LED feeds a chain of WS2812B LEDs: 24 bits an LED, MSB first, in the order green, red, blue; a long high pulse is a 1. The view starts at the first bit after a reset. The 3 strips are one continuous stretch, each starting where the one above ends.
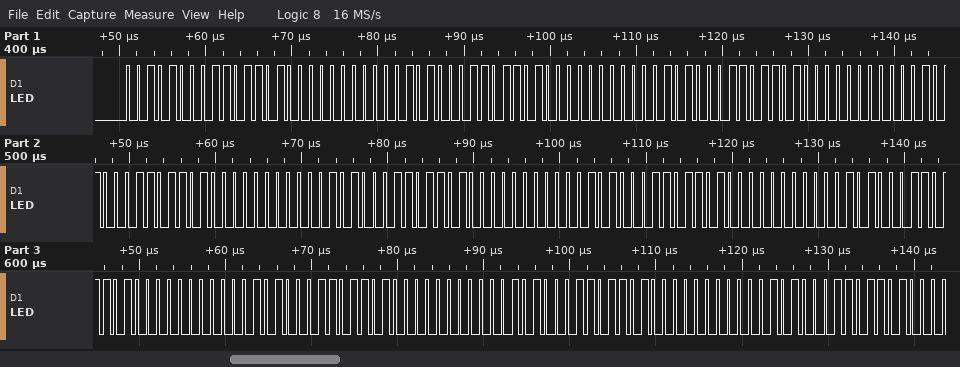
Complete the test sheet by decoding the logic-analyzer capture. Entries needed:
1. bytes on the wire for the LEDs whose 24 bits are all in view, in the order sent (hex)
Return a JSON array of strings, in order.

["28 DA 00 28 DA 00 28 DA 00 28 DA 00 28 DA 00 28 DA 00 28 DA 00 28 DA 00 28 DA 00"]
